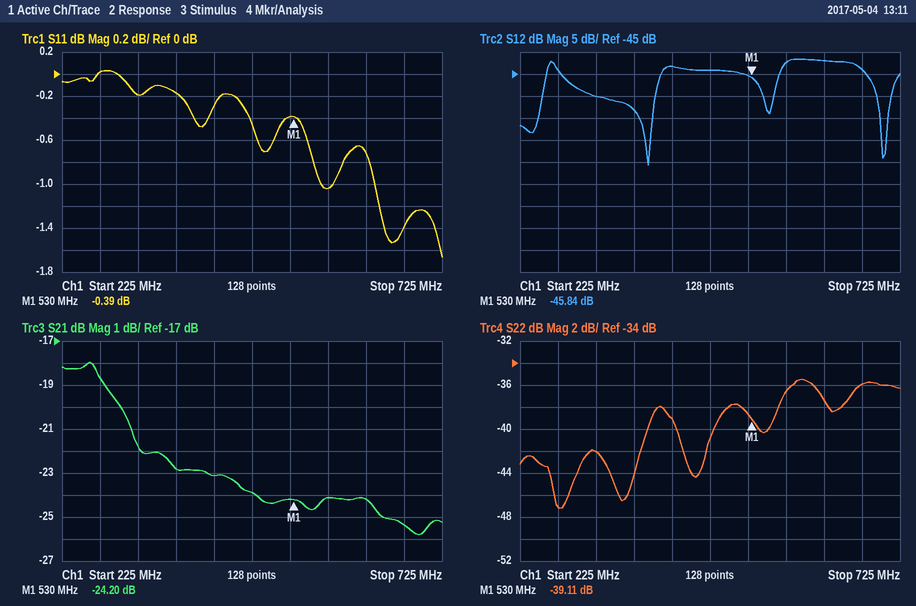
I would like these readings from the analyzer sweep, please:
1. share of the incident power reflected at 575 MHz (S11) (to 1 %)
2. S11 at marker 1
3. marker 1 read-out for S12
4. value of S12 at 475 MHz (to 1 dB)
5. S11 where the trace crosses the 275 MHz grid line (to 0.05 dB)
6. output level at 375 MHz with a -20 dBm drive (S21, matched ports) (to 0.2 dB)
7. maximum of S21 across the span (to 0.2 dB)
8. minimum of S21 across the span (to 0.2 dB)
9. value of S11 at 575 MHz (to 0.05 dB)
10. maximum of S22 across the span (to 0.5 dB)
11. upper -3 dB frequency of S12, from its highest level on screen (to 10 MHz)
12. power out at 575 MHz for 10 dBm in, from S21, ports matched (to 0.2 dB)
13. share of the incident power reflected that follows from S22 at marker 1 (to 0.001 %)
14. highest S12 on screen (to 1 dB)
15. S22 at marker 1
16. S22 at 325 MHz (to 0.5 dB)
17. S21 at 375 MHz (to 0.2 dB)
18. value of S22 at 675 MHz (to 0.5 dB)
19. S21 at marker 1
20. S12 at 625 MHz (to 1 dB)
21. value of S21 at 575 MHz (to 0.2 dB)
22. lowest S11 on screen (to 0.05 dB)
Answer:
79 %
-0.39 dB
-45.84 dB
-44 dB
0.00 dB
-42.8 dBm
-18.0 dB
-25.8 dB
-1.05 dB
-35.5 dB
680 MHz
-14.2 dBm
0.012 %
-42 dB
-39.11 dB
-42.0 dB
-22.8 dB
-36.0 dB
-24.20 dB
-42 dB
-24.2 dB
-1.65 dB
